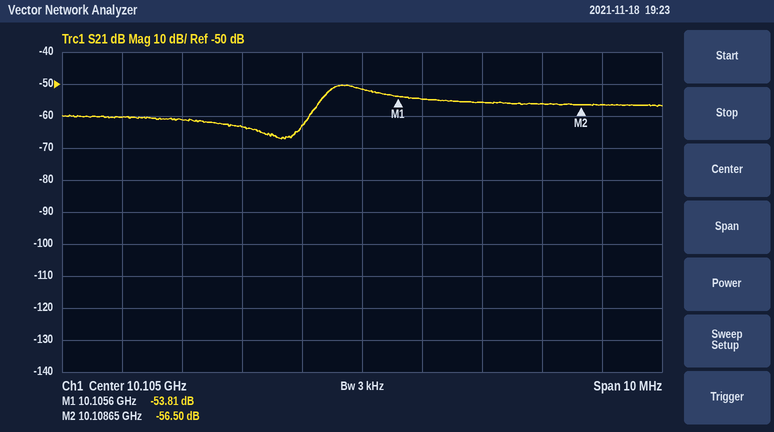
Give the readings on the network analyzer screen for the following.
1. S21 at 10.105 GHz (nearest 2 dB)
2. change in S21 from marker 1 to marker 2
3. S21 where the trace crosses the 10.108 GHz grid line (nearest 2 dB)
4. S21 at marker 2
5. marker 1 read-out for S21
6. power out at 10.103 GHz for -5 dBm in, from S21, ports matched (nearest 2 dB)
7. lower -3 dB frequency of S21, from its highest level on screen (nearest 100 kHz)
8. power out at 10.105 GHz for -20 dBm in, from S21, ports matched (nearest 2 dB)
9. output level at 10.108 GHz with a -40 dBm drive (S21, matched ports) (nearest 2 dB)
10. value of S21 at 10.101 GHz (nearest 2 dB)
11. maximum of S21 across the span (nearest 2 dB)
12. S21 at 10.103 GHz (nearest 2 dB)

-52 dB
-2.69 dB
-56 dB
-56.50 dB
-53.81 dB
-68 dBm
10.1044 GHz
-72 dBm
-96 dBm
-60 dB
-50 dB
-64 dB
